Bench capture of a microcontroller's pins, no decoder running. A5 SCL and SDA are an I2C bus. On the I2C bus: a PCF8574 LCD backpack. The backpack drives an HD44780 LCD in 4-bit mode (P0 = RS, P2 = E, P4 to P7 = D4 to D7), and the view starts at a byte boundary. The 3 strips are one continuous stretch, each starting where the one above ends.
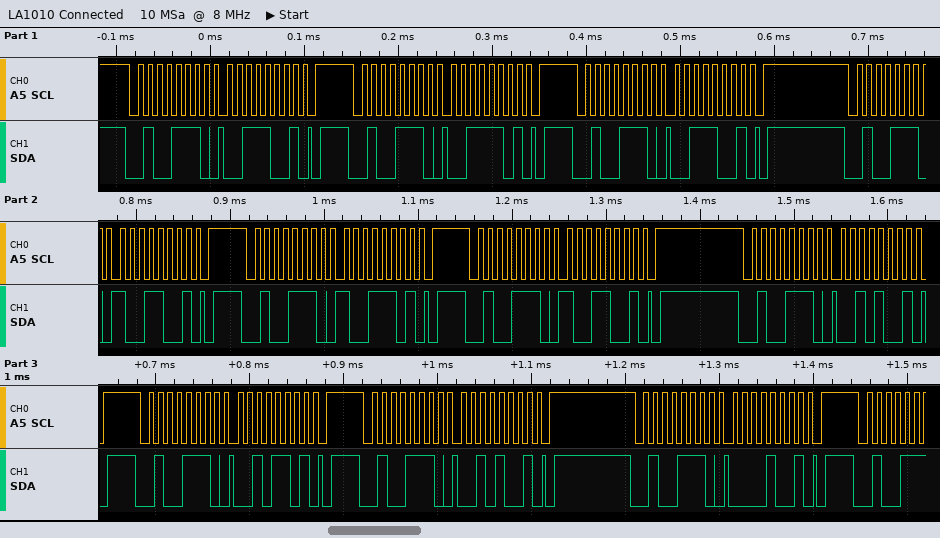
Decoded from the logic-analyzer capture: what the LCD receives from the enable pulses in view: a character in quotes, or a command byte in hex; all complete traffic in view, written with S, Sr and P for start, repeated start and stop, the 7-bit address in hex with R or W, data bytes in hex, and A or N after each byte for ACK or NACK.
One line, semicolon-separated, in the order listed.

'9'; S 27W A 39 A P S 27W A 3D A P S 27W A 39 A P S 27W A 99 A P S 27W A 9D A P S 27W A 99 A P S 27W A 29 A P S 27W A 2D A P S 27W A 29 A P S 27W A 09 A P
